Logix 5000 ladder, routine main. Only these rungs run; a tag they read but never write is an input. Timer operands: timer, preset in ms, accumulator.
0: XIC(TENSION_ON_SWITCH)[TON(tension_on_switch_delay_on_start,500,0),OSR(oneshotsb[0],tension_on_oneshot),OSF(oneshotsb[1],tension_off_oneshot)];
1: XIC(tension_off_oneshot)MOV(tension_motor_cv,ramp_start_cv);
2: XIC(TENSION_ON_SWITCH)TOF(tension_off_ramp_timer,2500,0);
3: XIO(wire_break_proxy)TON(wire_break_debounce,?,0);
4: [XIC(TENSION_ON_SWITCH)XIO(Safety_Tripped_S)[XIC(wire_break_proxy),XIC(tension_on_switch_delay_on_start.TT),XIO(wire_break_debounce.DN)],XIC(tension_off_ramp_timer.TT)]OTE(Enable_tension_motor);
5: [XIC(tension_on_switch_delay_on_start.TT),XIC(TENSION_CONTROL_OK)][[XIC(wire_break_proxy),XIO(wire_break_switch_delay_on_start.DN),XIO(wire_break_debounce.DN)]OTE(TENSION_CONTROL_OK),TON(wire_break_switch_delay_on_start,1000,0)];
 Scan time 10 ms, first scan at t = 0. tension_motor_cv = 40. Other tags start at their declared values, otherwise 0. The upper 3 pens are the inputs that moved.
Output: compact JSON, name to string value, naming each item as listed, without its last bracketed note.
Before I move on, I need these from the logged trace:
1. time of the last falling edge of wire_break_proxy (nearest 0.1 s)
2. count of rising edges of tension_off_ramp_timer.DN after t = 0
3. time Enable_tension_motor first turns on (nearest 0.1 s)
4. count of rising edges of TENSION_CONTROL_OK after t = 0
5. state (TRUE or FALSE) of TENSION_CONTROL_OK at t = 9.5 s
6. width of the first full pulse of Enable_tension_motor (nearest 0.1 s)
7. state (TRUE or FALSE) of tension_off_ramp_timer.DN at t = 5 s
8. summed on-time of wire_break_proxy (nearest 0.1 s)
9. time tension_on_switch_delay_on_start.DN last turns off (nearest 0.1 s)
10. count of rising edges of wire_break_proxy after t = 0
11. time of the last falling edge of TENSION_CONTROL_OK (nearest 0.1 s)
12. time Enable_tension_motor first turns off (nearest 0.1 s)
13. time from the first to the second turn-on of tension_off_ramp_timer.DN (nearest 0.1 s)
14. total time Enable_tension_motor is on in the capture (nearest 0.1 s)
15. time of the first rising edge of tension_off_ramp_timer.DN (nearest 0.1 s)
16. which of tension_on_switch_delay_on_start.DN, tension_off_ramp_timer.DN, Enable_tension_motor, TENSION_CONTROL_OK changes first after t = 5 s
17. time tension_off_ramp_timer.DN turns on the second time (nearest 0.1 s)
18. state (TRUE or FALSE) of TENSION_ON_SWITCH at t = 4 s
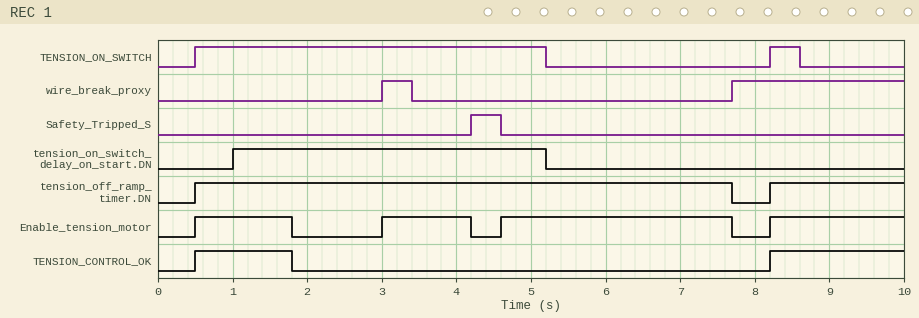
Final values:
{"time of the last falling edge of wire_break_proxy": "3.4 s", "count of rising edges of tension_off_ramp_timer.DN after t = 0": "2", "time Enable_tension_motor first turns on": "0.5 s", "count of rising edges of TENSION_CONTROL_OK after t = 0": "2", "state (TRUE or FALSE) of TENSION_CONTROL_OK at t = 9.5 s": "TRUE", "width of the first full pulse of Enable_tension_motor": "1.3 s", "state (TRUE or FALSE) of tension_off_ramp_timer.DN at t = 5 s": "TRUE", "summed on-time of wire_break_proxy": "2.7 s", "time tension_on_switch_delay_on_start.DN last turns off": "5.2 s", "count of rising edges of wire_break_proxy after t = 0": "2", "time of the last falling edge of TENSION_CONTROL_OK": "1.8 s", "time Enable_tension_motor first turns off": "1.8 s", "time from the first to the second turn-on of tension_off_ramp_timer.DN": "7.7 s", "total time Enable_tension_motor is on in the capture": "7.4 s", "time of the first rising edge of tension_off_ramp_timer.DN": "0.5 s", "which of tension_on_switch_delay_on_start.DN, tension_off_ramp_timer.DN, Enable_tension_motor, TENSION_CONTROL_OK changes first after t = 5 s": "tension_on_switch_delay_on_start.DN", "time tension_off_ramp_timer.DN turns on the second time": "8.2 s", "state (TRUE or FALSE) of TENSION_ON_SWITCH at t = 4 s": "TRUE"}
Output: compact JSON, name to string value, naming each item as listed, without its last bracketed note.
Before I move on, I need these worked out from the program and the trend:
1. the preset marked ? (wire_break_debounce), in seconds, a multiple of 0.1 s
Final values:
{"the preset marked ? (wire_break_debounce), in seconds, a multiple of 0.1 s": "1.8 s"}
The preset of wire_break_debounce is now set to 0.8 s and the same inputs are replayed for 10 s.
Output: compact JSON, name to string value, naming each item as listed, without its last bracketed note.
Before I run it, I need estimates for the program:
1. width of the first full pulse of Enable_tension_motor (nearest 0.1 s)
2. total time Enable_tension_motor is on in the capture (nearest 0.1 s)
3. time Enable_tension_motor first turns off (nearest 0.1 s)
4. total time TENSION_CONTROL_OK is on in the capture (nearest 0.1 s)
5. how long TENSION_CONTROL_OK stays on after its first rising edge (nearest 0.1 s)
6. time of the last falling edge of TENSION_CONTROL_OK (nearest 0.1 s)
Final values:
{"width of the first full pulse of Enable_tension_motor": "0.5 s", "total time Enable_tension_motor is on in the capture": "6.0 s", "time Enable_tension_motor first turns off": "1.0 s", "total time TENSION_CONTROL_OK is on in the capture": "2.8 s", "how long TENSION_CONTROL_OK stays on after its first rising edge": "1.0 s", "time of the last falling edge of TENSION_CONTROL_OK": "1.5 s"}
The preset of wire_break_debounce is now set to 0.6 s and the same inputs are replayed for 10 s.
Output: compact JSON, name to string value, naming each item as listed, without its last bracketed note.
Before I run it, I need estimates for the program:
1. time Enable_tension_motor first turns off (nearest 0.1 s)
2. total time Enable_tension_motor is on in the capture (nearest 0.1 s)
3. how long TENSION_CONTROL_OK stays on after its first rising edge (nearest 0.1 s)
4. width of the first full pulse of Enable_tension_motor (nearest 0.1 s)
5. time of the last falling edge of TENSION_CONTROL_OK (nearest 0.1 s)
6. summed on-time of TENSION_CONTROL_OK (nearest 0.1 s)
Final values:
{"time Enable_tension_motor first turns off": "1.0 s", "total time Enable_tension_motor is on in the capture": "5.8 s", "how long TENSION_CONTROL_OK stays on after its first rising edge": "1.0 s", "width of the first full pulse of Enable_tension_motor": "0.5 s", "time of the last falling edge of TENSION_CONTROL_OK": "1.5 s", "summed on-time of TENSION_CONTROL_OK": "2.8 s"}
